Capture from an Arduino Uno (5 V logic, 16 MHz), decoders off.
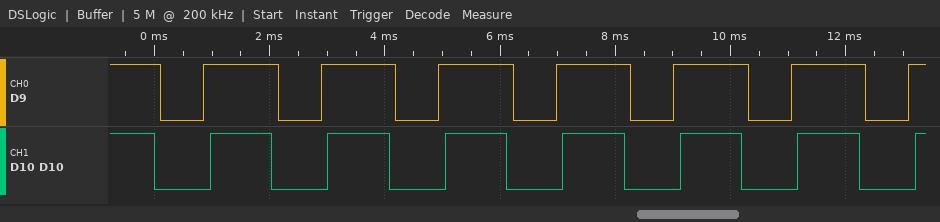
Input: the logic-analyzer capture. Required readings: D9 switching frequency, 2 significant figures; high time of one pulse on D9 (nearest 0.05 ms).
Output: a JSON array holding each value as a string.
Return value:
["490 Hz", "1.30 ms"]
